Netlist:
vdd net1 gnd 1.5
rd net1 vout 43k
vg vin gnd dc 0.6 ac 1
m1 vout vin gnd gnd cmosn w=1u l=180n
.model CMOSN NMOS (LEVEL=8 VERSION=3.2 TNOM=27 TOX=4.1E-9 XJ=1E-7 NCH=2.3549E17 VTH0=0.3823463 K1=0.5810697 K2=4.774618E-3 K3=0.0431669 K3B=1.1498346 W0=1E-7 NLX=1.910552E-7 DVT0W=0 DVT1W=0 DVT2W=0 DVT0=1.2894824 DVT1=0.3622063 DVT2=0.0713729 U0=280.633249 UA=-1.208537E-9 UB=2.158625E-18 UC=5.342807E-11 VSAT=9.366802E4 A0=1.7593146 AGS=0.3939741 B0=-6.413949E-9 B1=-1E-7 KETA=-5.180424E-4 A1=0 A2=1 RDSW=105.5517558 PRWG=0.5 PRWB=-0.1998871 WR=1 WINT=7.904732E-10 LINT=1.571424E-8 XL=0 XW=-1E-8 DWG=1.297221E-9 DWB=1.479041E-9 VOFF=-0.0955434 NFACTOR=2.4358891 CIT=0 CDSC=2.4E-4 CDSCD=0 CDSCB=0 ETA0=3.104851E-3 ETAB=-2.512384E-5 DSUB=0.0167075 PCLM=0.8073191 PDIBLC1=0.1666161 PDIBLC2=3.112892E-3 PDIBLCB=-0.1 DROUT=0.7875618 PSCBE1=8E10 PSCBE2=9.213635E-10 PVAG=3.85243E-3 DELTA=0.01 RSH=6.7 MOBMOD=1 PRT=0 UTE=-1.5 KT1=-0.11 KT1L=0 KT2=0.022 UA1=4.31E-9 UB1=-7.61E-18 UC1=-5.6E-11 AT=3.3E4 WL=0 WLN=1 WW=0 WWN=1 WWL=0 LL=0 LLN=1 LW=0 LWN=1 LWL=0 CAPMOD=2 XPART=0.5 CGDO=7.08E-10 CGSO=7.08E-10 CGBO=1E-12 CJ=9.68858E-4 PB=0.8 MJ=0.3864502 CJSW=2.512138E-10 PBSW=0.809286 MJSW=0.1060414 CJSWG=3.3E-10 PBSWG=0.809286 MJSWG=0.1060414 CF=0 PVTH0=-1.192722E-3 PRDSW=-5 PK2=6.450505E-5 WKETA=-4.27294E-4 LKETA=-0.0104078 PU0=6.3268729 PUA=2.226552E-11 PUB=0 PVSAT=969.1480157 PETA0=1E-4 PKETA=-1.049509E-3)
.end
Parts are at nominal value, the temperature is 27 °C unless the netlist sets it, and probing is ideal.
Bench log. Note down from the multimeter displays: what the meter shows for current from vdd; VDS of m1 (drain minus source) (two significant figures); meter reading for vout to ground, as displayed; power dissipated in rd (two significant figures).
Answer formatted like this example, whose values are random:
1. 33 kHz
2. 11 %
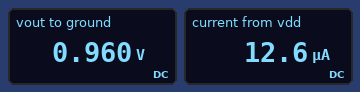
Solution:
1. 12.6 µA
2. 960 mV
3. 0.960 V
4. 6.8 µW
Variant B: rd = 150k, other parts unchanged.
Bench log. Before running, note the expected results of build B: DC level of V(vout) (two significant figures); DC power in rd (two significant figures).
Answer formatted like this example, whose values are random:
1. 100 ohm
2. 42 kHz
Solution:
1. 190 mV
2. 11 µW
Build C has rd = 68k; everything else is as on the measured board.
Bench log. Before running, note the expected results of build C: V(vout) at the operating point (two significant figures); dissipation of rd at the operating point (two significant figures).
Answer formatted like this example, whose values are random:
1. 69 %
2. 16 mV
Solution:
1. 720 mV
2. 8.9 µW
